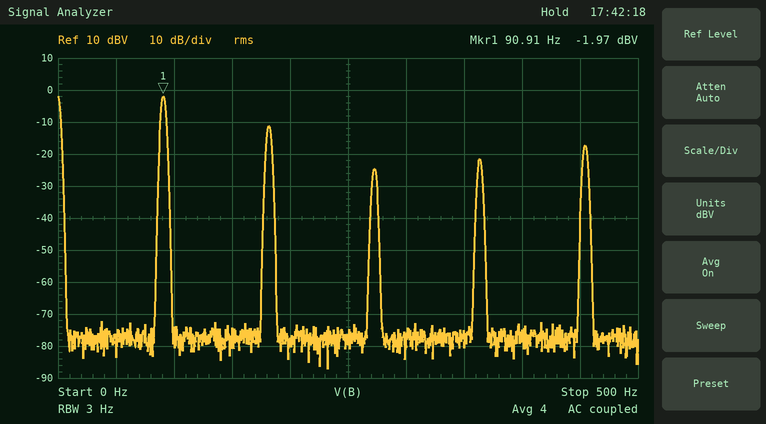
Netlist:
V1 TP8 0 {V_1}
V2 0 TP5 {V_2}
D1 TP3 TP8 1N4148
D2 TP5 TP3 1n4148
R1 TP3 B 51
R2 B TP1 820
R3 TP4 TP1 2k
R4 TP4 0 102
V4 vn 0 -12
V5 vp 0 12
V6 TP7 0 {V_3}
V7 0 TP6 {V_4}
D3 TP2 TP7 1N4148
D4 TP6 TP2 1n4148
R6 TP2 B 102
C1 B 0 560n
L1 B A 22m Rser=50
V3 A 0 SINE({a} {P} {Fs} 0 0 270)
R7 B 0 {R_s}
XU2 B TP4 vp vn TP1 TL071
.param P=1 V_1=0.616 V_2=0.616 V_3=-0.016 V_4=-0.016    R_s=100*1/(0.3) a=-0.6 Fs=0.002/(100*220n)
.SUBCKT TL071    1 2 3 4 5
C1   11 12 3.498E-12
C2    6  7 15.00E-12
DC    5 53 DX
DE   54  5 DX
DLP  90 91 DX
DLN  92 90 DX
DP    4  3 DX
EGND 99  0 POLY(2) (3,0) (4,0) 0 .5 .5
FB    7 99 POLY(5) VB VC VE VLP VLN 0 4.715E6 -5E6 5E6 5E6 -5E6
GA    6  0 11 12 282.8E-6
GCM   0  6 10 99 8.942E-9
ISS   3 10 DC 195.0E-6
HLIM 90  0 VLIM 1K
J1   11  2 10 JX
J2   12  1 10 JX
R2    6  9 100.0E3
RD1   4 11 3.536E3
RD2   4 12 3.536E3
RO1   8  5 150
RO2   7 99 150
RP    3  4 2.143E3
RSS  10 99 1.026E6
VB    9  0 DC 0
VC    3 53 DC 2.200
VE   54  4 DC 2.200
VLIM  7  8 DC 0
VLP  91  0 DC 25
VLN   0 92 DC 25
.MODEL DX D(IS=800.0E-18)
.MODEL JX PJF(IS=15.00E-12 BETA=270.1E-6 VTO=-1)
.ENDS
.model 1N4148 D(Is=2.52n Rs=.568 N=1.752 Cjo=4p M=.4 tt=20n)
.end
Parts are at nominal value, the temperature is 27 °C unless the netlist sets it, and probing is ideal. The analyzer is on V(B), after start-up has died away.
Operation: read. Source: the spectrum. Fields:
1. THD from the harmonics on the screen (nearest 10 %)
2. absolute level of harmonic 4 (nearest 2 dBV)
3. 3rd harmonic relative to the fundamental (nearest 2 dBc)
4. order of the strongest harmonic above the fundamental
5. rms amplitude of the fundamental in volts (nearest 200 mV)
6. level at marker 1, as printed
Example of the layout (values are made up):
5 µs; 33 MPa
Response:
40 %; -22 dBV; -22 dBc; 2; 800 mV; -1.97 dBV
